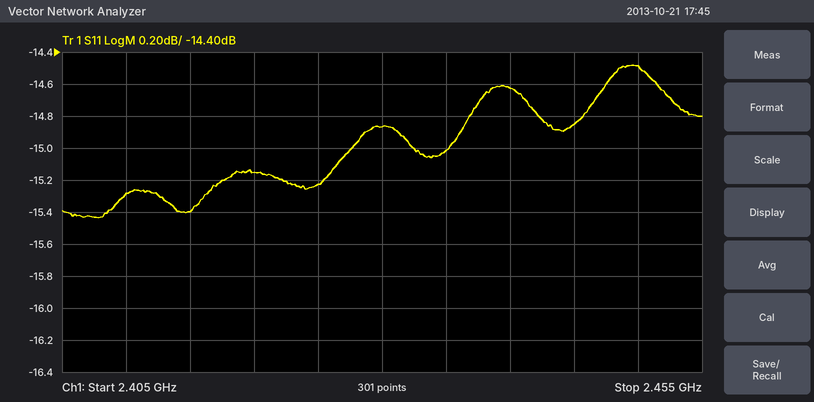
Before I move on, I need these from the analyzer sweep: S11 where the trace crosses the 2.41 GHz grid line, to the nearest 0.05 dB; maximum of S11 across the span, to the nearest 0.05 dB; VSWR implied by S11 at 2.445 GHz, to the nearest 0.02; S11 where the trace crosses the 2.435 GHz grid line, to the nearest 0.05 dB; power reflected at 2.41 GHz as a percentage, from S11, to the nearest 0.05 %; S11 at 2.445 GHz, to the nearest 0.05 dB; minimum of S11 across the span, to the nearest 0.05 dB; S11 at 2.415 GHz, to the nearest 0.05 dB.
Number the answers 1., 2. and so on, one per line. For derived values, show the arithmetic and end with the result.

1. -15.30 dB
2. -14.50 dB
3. |Γ| = 10^(-14.85/20) = 0.1809; VSWR = (1 + 0.1809)/(1 − 0.1809) ≈ 1.44
4. -15.00 dB
5. 10^(-15.3/10) ≈ 2.95 %
6. -14.85 dB
7. -15.45 dB
8. -15.40 dB
